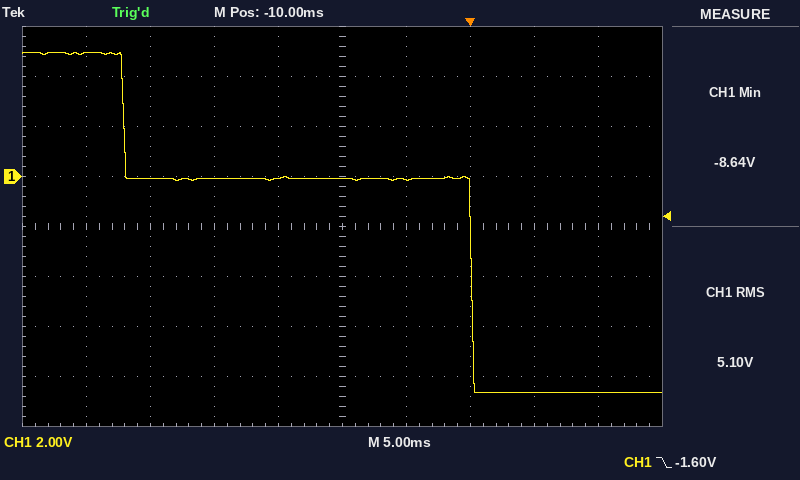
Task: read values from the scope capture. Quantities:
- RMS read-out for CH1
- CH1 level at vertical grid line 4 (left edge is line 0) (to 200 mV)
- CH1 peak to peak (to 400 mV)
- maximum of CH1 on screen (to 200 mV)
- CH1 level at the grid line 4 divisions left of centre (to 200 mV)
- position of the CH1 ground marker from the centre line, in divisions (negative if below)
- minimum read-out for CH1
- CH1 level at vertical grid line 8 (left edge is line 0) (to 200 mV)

5.10 V
0.0 V
13.6 V
5.0 V
5.0 V
+1.0 div
-8.64 V
-8.6 V
